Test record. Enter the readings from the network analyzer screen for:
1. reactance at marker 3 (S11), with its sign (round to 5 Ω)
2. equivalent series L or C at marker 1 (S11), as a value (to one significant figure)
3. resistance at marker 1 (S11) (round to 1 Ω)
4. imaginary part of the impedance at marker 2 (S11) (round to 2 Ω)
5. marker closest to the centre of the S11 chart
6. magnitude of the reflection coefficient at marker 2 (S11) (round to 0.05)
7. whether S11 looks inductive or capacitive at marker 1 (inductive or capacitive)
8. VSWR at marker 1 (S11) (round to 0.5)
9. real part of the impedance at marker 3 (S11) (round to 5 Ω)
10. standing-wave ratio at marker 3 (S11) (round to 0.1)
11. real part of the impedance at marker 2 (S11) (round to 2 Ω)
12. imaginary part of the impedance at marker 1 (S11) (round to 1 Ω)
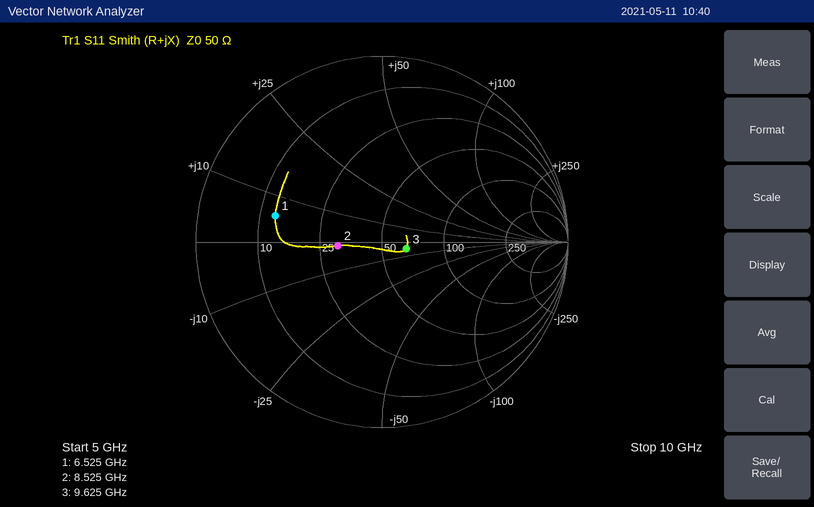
-5 Ω
100 pH
13 Ω
-2 Ω
marker 3
0.25
inductive
4.0
65 Ω
1.3
30 Ω
+6 Ω
